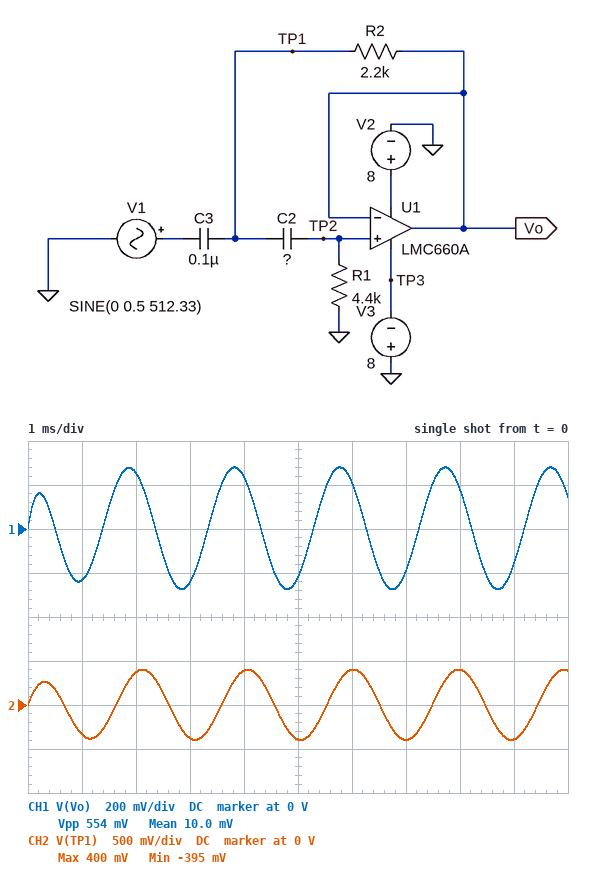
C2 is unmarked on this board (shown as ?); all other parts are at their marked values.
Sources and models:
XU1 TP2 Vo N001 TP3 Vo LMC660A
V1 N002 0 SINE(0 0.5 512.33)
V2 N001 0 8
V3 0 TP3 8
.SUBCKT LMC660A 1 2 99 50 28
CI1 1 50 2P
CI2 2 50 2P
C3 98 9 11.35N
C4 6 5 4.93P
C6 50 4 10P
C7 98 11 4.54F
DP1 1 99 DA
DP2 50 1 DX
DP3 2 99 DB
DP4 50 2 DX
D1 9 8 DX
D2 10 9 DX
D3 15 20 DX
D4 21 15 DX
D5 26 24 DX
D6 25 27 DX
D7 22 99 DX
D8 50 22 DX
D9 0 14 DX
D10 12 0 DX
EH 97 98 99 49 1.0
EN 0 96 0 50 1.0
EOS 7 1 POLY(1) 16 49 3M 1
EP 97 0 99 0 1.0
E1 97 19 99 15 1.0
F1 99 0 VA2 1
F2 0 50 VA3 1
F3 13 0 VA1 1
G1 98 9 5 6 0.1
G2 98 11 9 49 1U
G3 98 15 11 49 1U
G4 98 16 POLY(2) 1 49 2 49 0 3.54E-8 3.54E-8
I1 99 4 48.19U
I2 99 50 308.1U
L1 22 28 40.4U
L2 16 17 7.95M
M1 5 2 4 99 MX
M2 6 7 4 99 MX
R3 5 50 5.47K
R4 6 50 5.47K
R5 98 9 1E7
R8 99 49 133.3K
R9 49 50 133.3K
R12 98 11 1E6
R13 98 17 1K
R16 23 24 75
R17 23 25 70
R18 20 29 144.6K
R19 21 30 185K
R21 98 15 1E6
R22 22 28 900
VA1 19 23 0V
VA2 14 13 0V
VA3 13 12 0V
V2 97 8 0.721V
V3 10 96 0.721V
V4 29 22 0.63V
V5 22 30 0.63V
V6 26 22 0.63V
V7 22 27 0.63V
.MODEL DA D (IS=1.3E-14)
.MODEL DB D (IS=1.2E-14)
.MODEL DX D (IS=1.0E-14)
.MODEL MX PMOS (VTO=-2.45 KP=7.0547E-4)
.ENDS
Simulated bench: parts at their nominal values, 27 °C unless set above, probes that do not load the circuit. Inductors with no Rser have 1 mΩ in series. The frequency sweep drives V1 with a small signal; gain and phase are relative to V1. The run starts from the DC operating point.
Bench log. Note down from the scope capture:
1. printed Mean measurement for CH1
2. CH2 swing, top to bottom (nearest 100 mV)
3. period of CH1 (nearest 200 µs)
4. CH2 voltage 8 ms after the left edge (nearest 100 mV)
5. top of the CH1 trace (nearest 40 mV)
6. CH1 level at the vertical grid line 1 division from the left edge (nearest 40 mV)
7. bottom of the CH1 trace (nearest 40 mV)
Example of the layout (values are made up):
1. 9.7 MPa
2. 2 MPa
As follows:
1. 10.0 mV
2. 800 mV
3. 2.0 ms
4. 400 mV
5. 280 mV
6. -240 mV
7. -280 mV
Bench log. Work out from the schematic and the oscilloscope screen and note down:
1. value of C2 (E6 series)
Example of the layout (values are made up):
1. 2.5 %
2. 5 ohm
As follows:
1. 68 nF
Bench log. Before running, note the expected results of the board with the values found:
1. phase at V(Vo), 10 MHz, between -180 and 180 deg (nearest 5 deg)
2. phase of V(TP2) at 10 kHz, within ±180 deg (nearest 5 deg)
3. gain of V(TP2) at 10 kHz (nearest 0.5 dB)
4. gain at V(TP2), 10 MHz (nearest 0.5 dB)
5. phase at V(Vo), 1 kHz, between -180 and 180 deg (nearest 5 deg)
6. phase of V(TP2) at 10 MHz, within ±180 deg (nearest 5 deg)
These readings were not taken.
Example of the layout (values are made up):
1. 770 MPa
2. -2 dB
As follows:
1. 10 deg
2. 5 deg
3. 0 dB
4. 0 dB
5. 55 deg
6. 0 deg
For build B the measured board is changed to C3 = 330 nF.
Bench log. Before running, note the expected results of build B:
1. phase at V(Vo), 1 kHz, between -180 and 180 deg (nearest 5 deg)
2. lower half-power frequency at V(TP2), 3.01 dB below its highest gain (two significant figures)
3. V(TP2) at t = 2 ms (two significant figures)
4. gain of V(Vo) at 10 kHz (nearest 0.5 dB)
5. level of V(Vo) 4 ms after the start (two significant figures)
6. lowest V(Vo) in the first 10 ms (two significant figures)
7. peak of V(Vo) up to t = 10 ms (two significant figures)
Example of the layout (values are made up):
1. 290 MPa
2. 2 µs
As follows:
1. 35 deg
2. 490 Hz
3. 360 mV
4. 0 dB
5. 370 mV
6. -360 mV
7. 380 mV
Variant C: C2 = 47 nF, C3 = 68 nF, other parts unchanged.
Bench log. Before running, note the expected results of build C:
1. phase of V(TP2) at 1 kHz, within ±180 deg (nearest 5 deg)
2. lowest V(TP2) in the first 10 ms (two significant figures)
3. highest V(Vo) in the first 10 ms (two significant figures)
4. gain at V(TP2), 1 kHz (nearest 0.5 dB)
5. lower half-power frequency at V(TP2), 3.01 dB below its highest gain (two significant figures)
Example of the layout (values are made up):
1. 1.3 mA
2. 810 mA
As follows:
1. 80 deg
2. -150 mV
3. 150 mV
4. -2.5 dB
5. 920 Hz
